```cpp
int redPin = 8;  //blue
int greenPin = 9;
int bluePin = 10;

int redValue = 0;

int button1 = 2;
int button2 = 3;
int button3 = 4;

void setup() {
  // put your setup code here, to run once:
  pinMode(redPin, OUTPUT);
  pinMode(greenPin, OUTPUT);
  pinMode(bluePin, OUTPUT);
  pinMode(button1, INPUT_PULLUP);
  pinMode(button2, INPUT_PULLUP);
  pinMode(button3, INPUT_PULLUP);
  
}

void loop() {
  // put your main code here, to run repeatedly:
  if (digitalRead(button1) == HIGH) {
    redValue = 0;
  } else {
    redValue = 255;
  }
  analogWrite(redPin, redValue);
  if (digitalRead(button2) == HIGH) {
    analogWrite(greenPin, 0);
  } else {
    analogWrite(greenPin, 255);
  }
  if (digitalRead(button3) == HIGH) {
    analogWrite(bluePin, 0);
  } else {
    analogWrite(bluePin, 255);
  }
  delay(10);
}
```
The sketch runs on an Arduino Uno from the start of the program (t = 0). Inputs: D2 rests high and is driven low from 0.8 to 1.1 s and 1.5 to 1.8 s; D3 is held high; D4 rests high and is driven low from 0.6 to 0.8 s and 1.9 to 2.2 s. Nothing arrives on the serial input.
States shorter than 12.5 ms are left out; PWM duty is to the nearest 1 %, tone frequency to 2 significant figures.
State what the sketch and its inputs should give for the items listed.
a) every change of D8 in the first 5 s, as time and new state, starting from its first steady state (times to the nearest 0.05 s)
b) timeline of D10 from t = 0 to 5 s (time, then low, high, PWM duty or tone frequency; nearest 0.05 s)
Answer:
0 s low; 0.8 s high; 1.1 s low; 1.5 s high; 1.8 s low
0 s low; 0.6 s high; 0.8 s low; 1.9 s high; 2.2 s low
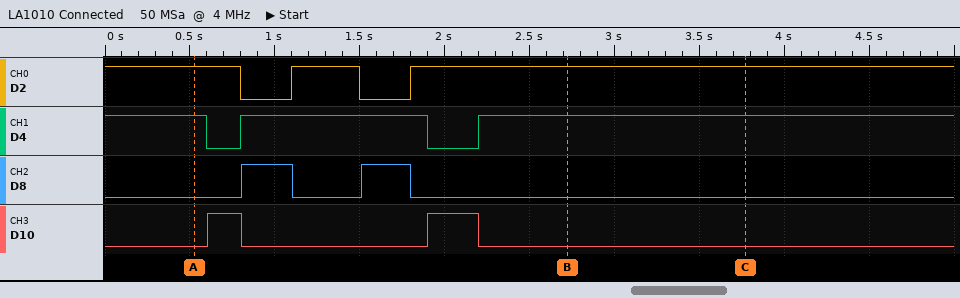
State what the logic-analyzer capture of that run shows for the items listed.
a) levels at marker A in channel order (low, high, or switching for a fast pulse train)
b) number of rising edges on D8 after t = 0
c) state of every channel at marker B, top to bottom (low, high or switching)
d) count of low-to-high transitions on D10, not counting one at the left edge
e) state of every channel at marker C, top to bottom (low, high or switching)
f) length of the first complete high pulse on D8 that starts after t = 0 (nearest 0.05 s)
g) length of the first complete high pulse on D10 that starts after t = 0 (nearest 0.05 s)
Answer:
D2 high, D4 high, D8 low, D10 low
2
D2 high, D4 high, D8 low, D10 low
2
D2 high, D4 high, D8 low, D10 low
0.30 s
0.20 s
